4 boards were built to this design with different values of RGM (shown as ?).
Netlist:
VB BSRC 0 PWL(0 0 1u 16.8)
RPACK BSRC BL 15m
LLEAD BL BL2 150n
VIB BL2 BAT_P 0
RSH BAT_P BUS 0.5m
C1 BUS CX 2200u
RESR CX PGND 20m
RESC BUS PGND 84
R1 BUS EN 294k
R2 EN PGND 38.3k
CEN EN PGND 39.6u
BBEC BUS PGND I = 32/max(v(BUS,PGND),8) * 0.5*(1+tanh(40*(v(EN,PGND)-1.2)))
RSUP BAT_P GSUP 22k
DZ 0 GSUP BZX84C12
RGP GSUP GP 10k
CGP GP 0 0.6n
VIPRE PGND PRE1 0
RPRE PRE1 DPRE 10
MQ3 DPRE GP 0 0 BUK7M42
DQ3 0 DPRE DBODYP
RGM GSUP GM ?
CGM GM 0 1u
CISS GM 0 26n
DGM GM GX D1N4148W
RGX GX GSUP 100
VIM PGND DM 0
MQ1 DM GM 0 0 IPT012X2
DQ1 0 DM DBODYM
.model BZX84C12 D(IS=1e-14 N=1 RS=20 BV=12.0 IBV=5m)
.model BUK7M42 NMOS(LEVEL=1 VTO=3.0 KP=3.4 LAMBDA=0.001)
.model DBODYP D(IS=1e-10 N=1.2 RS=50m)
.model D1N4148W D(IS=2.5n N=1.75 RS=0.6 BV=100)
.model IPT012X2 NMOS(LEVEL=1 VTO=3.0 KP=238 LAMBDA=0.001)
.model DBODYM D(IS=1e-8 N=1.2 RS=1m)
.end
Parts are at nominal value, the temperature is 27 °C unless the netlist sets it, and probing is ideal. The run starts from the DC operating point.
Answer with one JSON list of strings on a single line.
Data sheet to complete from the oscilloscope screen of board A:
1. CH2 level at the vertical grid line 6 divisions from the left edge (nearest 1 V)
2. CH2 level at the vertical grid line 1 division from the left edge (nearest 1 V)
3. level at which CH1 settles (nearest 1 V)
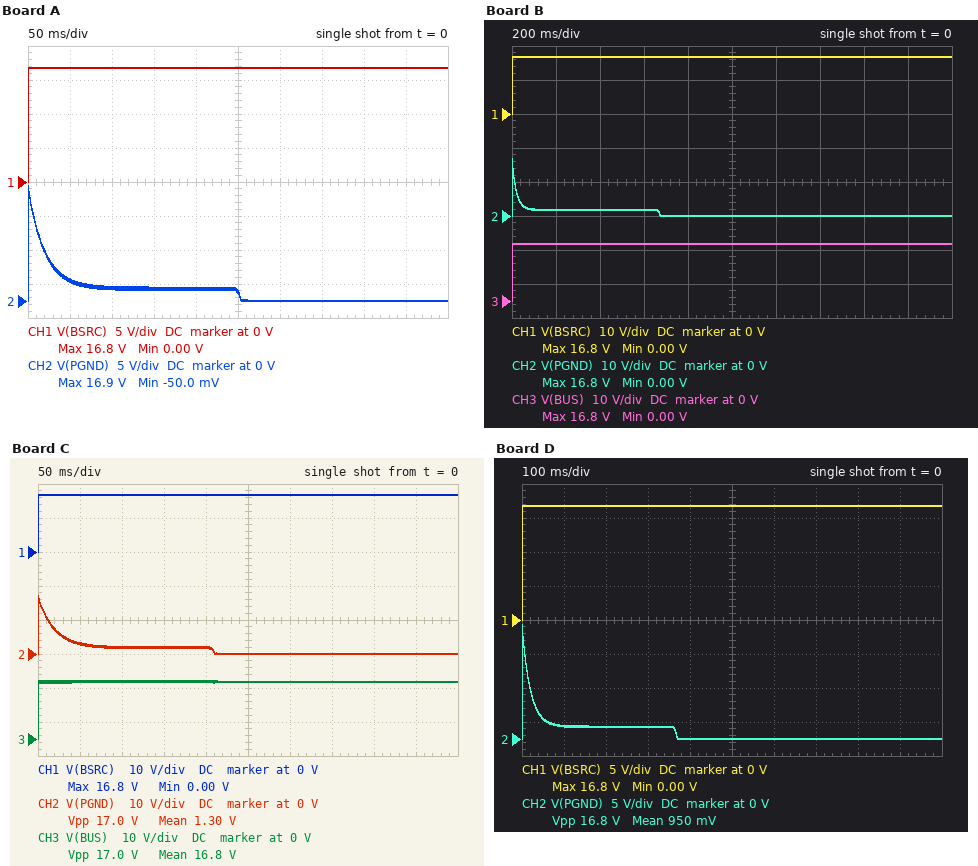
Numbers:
["0 V", "3 V", "17 V"]
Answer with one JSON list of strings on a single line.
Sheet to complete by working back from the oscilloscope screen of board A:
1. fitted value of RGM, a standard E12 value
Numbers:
["820 kΩ"]
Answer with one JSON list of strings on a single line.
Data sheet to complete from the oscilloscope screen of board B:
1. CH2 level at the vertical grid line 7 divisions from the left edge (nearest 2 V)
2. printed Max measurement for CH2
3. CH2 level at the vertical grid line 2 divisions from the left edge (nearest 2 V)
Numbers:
["0 V", "16.8 V", "2 V"]
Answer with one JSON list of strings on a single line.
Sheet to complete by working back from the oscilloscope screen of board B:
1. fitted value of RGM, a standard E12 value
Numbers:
["2.2 MΩ"]
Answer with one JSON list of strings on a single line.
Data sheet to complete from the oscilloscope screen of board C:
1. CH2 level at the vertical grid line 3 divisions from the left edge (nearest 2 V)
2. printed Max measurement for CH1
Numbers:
["2 V", "16.8 V"]
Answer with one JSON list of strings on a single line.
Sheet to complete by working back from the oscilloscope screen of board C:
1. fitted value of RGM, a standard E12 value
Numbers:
["680 kΩ"]
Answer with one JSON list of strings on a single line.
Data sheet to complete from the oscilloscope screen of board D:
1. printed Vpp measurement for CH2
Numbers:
["16.8 V"]
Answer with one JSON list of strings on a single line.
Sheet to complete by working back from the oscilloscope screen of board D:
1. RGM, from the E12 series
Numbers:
["1.2 MΩ"]
